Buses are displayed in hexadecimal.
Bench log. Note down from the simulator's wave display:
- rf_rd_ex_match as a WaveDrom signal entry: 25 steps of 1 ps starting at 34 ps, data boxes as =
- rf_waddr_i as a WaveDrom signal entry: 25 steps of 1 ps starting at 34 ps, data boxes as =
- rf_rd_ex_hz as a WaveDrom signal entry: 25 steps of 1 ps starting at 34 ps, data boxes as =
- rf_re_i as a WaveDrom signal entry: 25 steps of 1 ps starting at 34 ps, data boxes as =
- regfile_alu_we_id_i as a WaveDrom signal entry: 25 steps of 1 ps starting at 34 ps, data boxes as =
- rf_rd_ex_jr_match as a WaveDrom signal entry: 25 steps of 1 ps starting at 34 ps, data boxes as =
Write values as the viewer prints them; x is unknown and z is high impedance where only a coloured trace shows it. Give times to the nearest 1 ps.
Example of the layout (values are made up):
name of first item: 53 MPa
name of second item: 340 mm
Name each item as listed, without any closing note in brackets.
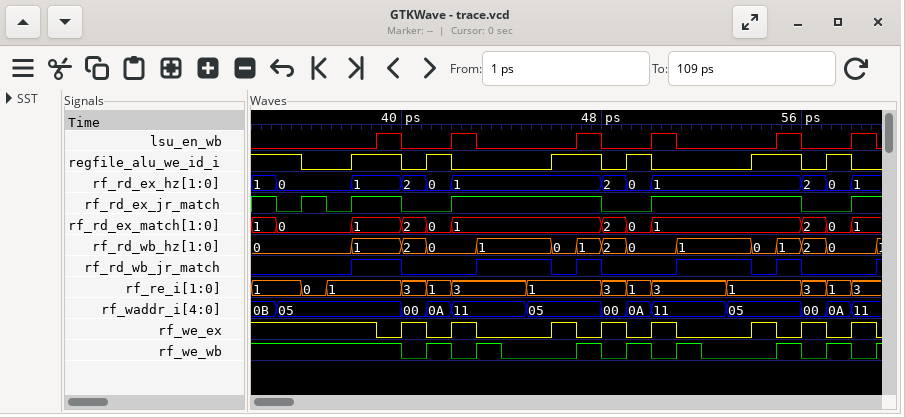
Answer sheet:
rf_rd_ex_match as a WaveDrom signal entry: 25 steps of 1 ps starting at 34 ps, data boxes as =: {name: 'rf_rd_ex_match', wave: '==..=.===.....===.....===', data: '1 0 1 2 0 1 2 0 1 2 0 1'}
rf_waddr_i as a WaveDrom signal entry: 25 steps of 1 ps starting at 34 ps, data boxes as =: {name: 'rf_waddr_i', wave: '==....===..=..===..=..===', data: '0B 05 00 0A 11 05 00 0A 11 05 00 0A 11'}
rf_rd_ex_hz as a WaveDrom signal entry: 25 steps of 1 ps starting at 34 ps, data boxes as =: {name: 'rf_rd_ex_hz', wave: '==..=.===.....===.....===', data: '1 0 1 2 0 1 2 0 1 2 0 1'}
rf_re_i as a WaveDrom signal entry: 25 steps of 1 ps starting at 34 ps, data boxes as =: {name: 'rf_re_i', wave: '=.==..===..=..===..=..===', data: '1 0 1 3 1 3 1 3 1 3 1 3 1 3'}
regfile_alu_we_id_i as a WaveDrom signal entry: 25 steps of 1 ps starting at 34 ps, data boxes as =: {name: 'regfile_alu_we_id_i', wave: '1.0.1.010...1.010...1.010'}
rf_rd_ex_jr_match as a WaveDrom signal entry: 25 steps of 1 ps starting at 34 ps, data boxes as =: {name: 'rf_rd_ex_jr_match', wave: '10101.0.1.....0.1.....0.1'}
